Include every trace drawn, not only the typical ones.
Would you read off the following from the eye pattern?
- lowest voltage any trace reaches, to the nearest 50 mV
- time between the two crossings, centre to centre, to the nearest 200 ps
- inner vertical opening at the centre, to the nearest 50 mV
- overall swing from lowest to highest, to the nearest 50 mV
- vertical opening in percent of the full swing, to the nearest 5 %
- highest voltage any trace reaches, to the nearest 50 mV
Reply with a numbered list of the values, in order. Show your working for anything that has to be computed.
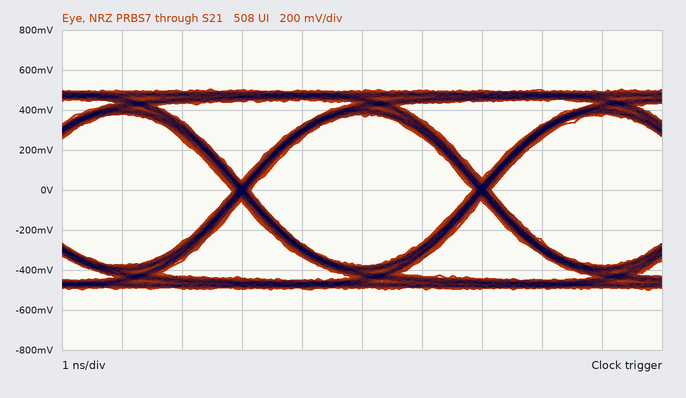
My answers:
1. -500 mV
2. 4.0 ns
3. 750 mV
4. 1.00 V
5. 750 mV / 1.00 V ≈ 75 %
6. 500 mV
